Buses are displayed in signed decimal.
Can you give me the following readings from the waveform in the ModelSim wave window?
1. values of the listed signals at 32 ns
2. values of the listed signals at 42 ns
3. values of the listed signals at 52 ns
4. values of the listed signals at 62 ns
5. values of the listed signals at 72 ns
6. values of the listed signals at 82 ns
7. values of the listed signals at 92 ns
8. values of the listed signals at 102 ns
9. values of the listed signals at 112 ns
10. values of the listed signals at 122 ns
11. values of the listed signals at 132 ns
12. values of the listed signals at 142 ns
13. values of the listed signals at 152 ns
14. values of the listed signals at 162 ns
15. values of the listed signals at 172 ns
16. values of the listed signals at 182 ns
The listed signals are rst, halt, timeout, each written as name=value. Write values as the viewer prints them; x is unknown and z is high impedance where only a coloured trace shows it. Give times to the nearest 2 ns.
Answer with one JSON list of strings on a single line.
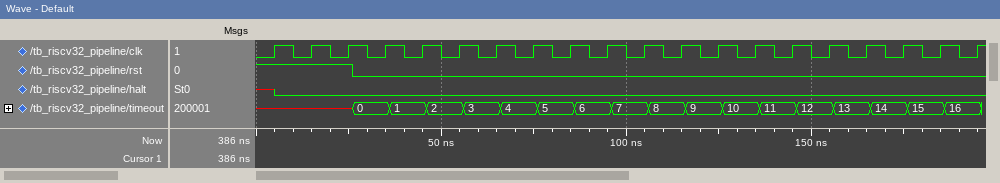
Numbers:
["rst=0, halt=0, timeout=0", "rst=0, halt=0, timeout=1", "rst=0, halt=0, timeout=2", "rst=0, halt=0, timeout=3", "rst=0, halt=0, timeout=4", "rst=0, halt=0, timeout=5", "rst=0, halt=0, timeout=6", "rst=0, halt=0, timeout=7", "rst=0, halt=0, timeout=8", "rst=0, halt=0, timeout=9", "rst=0, halt=0, timeout=10", "rst=0, halt=0, timeout=11", "rst=0, halt=0, timeout=12", "rst=0, halt=0, timeout=13", "rst=0, halt=0, timeout=14", "rst=0, halt=0, timeout=15"]
